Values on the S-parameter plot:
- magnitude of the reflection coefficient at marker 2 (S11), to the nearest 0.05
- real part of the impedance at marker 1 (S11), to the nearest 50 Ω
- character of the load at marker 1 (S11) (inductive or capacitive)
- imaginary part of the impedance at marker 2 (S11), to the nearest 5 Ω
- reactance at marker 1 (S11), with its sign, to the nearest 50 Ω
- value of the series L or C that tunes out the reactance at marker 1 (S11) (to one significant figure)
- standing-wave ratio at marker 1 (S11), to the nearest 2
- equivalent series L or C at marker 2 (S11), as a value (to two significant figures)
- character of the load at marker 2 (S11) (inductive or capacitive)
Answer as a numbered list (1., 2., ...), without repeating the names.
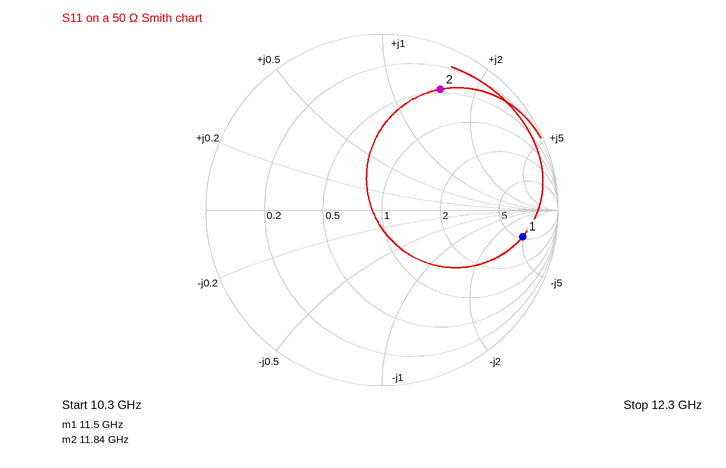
1. 0.75
2. 250 Ω
3. capacitive
4. +75 Ω
5. -250 Ω
6. 3 nH
7. 10
8. 1.0 nH
9. inductive
